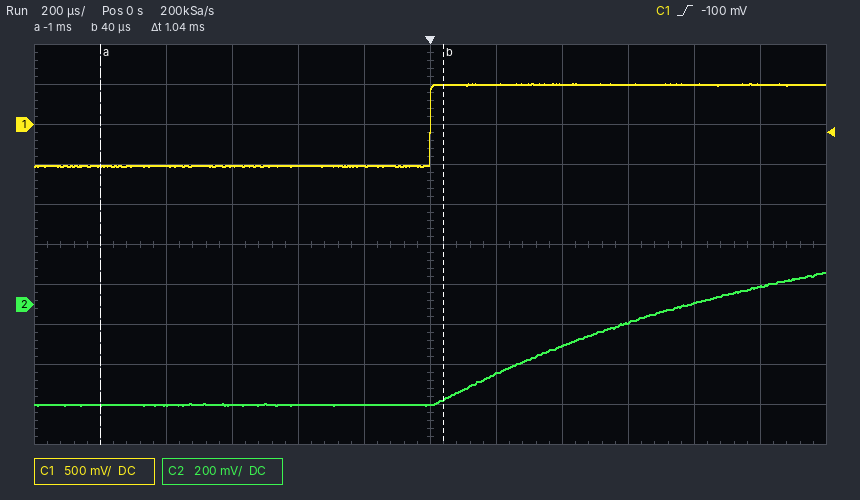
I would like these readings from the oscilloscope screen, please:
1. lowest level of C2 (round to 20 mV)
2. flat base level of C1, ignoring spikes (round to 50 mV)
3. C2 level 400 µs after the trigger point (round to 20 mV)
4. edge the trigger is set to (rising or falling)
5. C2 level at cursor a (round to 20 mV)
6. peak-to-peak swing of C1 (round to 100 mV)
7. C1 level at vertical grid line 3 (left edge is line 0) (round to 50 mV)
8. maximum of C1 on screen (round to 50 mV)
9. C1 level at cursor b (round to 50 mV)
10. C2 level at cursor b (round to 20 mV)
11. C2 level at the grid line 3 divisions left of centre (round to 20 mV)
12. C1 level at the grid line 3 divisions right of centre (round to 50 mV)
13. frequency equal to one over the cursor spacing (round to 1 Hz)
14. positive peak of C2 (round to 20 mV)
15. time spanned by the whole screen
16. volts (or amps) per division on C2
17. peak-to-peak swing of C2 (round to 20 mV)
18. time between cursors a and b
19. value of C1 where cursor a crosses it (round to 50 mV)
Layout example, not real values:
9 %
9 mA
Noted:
-500 mV
-500 mV
-200 mV
rising
-500 mV
1.00 V
-500 mV
500 mV
500 mV
-480 mV
-500 mV
500 mV
962 Hz
160 mV
2.4 ms
200 mV
660 mV
1.04 ms
-500 mV
